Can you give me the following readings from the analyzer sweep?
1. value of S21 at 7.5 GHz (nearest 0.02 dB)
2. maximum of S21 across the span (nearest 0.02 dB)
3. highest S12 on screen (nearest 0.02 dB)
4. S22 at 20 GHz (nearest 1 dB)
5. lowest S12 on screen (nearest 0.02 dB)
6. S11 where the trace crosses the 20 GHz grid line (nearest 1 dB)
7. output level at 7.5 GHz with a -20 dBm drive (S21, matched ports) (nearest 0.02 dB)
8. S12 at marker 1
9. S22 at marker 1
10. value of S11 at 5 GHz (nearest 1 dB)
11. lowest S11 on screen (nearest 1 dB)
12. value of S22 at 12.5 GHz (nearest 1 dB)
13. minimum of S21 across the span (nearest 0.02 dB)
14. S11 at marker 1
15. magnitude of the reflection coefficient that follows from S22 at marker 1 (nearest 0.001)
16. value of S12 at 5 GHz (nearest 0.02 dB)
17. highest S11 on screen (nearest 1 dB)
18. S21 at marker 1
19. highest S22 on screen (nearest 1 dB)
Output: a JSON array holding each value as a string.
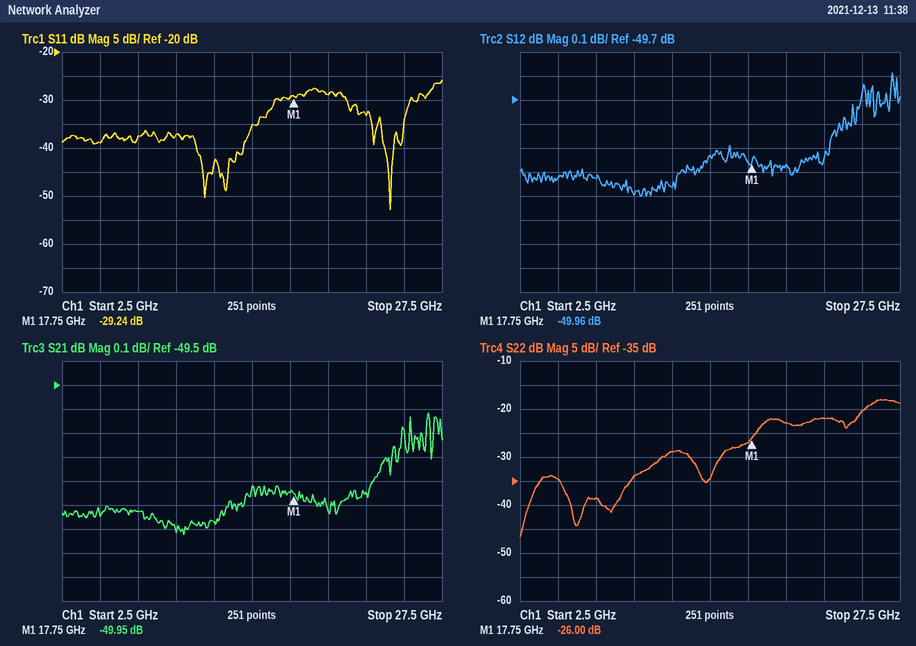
["-50.02 dB", "-49.62 dB", "-49.58 dB", "-23 dB", "-50.10 dB", "-29 dB", "-70.02 dBm", "-49.96 dB", "-26.00 dB", "-39 dB", "-53 dB", "-29 dB", "-50.12 dB", "-29.24 dB", "0.050", "-50.02 dB", "-26 dB", "-49.95 dB", "-18 dB"]
